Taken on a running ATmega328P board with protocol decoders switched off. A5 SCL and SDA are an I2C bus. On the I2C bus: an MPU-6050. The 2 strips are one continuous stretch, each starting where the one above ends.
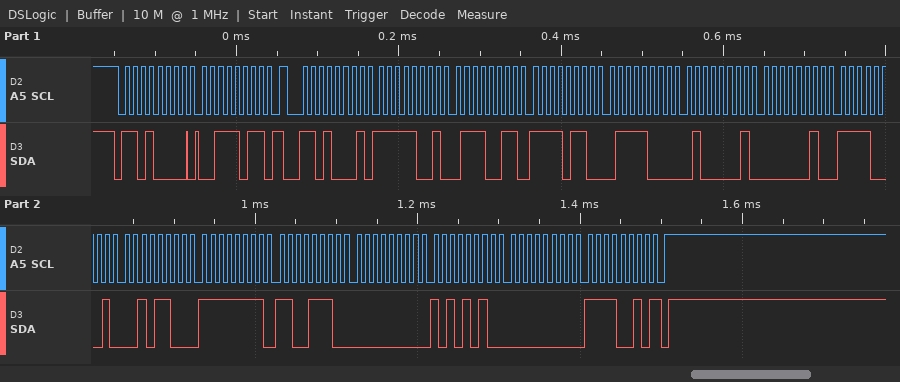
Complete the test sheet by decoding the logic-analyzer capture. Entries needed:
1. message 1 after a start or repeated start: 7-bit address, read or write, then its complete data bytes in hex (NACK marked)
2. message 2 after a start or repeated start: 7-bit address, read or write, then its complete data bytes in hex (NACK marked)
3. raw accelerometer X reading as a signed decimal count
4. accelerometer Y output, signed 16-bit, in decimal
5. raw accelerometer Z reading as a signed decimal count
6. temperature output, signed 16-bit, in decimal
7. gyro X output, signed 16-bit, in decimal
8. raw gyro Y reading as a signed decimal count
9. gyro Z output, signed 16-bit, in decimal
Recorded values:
0x68 write: 3B
0x68 read: F9 73 F6 78 41 02 F1 2C FF CE 00 AA 00 F2 NACK
-1677
-2440
16642
-3796
-50
170
242
